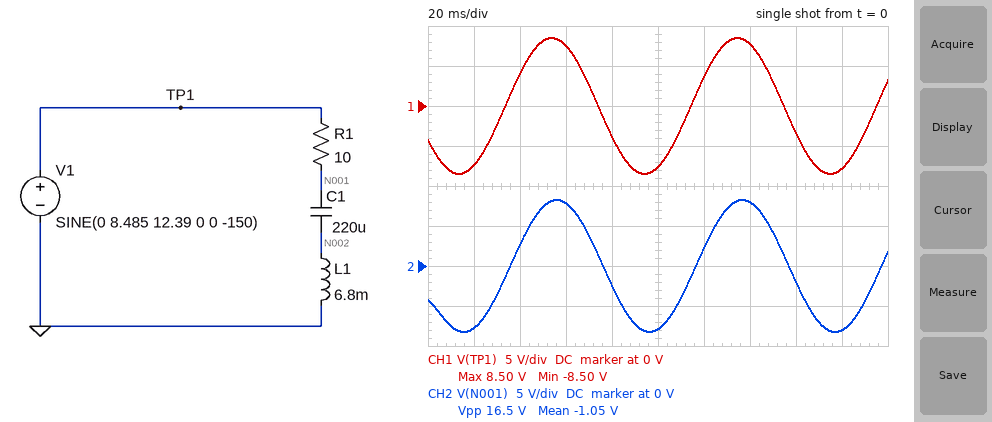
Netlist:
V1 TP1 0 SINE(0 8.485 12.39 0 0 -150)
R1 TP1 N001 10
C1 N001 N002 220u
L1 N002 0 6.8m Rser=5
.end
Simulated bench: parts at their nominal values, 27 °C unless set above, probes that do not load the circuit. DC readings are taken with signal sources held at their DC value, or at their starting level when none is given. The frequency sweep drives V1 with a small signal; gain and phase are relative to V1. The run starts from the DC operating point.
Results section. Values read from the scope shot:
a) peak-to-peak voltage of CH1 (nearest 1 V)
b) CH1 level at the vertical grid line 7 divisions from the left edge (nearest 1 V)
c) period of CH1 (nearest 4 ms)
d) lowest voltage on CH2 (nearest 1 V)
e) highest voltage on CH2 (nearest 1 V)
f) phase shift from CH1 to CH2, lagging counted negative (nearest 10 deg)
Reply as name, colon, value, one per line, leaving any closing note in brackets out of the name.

peak-to-peak voltage of CH1: 17 V
CH1 level at the vertical grid line 7 divisions from the left edge: 8 V
period of CH1: 80 ms
lowest voltage on CH2: -8 V
highest voltage on CH2: 8 V
phase shift from CH1 to CH2, lagging counted negative: -10 deg
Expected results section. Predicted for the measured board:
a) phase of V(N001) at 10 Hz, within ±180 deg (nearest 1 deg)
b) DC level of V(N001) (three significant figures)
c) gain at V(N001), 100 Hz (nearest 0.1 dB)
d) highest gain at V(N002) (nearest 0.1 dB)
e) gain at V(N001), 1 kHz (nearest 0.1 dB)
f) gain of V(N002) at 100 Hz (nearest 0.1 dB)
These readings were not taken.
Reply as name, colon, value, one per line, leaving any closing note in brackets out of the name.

phase of V(N001) at 10 Hz, within ±180 deg: -8 deg
DC level of V(N001): -4.24 V
gain at V(N001), 100 Hz: -8.4 dB
highest gain at V(N002): 0 dB
gain at V(N001), 1 kHz: -0.5 dB
gain of V(N002) at 100 Hz: -7.3 dB
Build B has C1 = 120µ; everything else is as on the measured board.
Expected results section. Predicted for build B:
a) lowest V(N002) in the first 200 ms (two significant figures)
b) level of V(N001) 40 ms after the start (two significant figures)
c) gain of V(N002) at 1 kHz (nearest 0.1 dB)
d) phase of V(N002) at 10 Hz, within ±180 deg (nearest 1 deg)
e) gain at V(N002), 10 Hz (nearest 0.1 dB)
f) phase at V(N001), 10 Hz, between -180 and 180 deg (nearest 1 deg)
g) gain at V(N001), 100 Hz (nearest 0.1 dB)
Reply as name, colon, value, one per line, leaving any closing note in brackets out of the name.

lowest V(N002) in the first 200 ms: -400 mV
level of V(N001) 40 ms after the start: 3.3 V
gain of V(N002) at 1 kHz: -0.2 dB
phase of V(N002) at 10 Hz, within ±180 deg: 88 deg
gain at V(N002), 10 Hz: -28.5 dB
phase at V(N001), 10 Hz, between -180 and 180 deg: -4 deg
gain at V(N001), 100 Hz: -4.6 dB
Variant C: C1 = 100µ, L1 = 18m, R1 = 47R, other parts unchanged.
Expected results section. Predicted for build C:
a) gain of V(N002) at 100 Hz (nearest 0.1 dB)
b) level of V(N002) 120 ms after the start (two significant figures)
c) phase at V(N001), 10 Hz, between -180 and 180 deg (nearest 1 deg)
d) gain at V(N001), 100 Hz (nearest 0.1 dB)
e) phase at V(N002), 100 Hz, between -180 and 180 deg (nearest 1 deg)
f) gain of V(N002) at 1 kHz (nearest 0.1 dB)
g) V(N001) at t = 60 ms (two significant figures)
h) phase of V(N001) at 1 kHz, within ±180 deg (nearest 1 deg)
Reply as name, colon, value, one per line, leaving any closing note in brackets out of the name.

gain of V(N002) at 100 Hz: -12.5 dB
level of V(N002) 120 ms after the start: 300 mV
phase at V(N001), 10 Hz, between -180 and 180 deg: -16 deg
gain at V(N001), 100 Hz: -17.7 dB
phase at V(N002), 100 Hz, between -180 and 180 deg: 71 deg
gain of V(N002) at 1 kHz: -0.7 dB
V(N001) at t = 60 ms: 7.8 V
phase of V(N001) at 1 kHz, within ±180 deg: 22 deg
